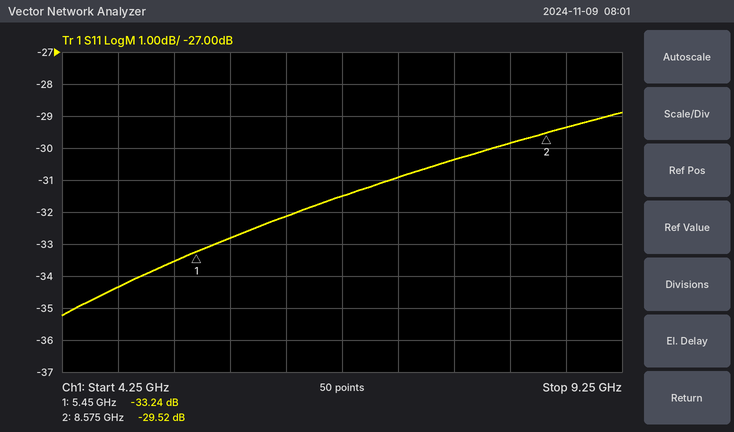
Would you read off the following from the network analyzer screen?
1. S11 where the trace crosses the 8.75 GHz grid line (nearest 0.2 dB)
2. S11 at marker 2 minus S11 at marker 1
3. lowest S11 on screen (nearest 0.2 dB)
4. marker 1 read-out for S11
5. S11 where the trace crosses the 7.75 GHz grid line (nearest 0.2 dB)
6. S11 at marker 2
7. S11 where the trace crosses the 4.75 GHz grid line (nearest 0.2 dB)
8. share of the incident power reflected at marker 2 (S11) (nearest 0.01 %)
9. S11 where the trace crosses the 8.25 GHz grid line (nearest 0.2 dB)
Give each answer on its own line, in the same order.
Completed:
-29.4 dB
3.72 dB
-35.2 dB
-33.24 dB
-30.4 dB
-29.52 dB
-34.4 dB
0.11 %
-29.8 dB
